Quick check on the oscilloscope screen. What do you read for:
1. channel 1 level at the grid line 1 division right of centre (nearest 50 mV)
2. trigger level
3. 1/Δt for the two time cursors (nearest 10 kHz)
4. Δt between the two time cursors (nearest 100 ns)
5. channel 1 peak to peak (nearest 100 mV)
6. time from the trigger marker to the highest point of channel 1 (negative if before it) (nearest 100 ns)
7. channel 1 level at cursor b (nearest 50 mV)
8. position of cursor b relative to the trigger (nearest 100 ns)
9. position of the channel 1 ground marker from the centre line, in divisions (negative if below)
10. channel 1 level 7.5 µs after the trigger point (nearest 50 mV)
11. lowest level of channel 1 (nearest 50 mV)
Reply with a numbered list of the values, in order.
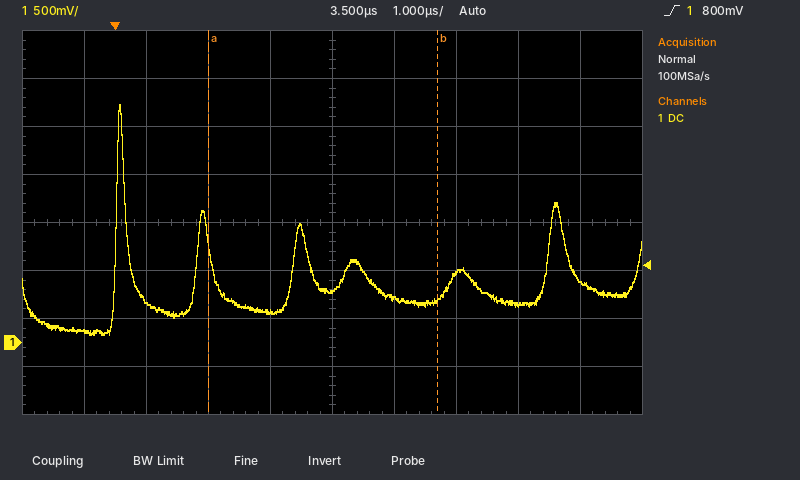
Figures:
1. 450 mV
2. 800 mV
3. 270 kHz
4. 3.7 µs
5. 2.40 V
6. +100 ns
7. 450 mV
8. +5.2 µs
9. -2.5 div
10. 650 mV
11. 100 mV
